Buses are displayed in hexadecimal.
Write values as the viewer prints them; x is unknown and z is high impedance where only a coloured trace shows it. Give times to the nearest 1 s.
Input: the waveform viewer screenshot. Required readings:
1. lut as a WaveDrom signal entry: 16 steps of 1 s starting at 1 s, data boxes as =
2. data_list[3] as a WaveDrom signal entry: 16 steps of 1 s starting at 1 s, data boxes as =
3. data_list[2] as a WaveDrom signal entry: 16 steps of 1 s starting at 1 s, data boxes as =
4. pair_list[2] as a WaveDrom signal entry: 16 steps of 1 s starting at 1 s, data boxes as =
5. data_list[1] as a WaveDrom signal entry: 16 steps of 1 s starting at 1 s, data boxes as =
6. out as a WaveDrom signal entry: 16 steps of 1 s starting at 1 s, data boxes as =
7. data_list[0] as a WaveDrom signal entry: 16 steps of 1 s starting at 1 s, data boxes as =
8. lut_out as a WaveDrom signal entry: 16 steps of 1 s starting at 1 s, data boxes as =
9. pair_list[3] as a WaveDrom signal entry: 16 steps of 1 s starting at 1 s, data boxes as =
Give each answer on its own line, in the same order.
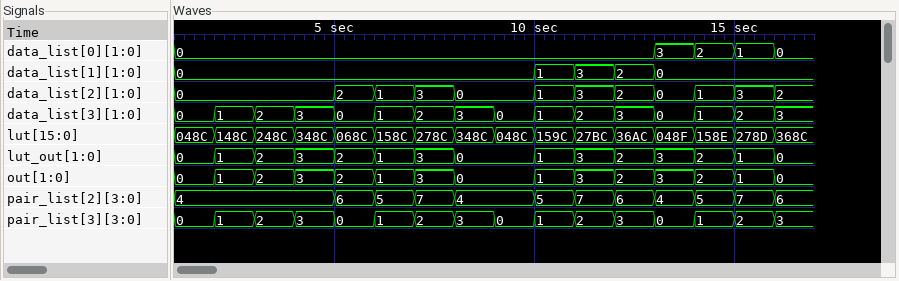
{name: 'lut', wave: '================', data: '048C 148C 248C 348C 068C 158C 278C 348C 048C 159C 27BC 36AC 048F 158E 278D 368C'}
{name: 'data_list[3]', wave: '================', data: '0 1 2 3 0 1 2 3 0 1 2 3 0 1 2 3'}
{name: 'data_list[2]', wave: '=...====.=======', data: '0 2 1 3 0 1 3 2 0 1 3 2'}
{name: 'pair_list[2]', wave: '=...====.=======', data: '4 6 5 7 4 5 7 6 4 5 7 6'}
{name: 'data_list[1]', wave: '=........====...', data: '0 1 3 2 0'}
{name: 'out', wave: '========.=======', data: '0 1 2 3 2 1 3 0 1 3 2 3 2 1 0'}
{name: 'data_list[0]', wave: '=...........====', data: '0 3 2 1 0'}
{name: 'lut_out', wave: '========.=======', data: '0 1 2 3 2 1 3 0 1 3 2 3 2 1 0'}
{name: 'pair_list[3]', wave: '================', data: '0 1 2 3 0 1 2 3 0 1 2 3 0 1 2 3'}
